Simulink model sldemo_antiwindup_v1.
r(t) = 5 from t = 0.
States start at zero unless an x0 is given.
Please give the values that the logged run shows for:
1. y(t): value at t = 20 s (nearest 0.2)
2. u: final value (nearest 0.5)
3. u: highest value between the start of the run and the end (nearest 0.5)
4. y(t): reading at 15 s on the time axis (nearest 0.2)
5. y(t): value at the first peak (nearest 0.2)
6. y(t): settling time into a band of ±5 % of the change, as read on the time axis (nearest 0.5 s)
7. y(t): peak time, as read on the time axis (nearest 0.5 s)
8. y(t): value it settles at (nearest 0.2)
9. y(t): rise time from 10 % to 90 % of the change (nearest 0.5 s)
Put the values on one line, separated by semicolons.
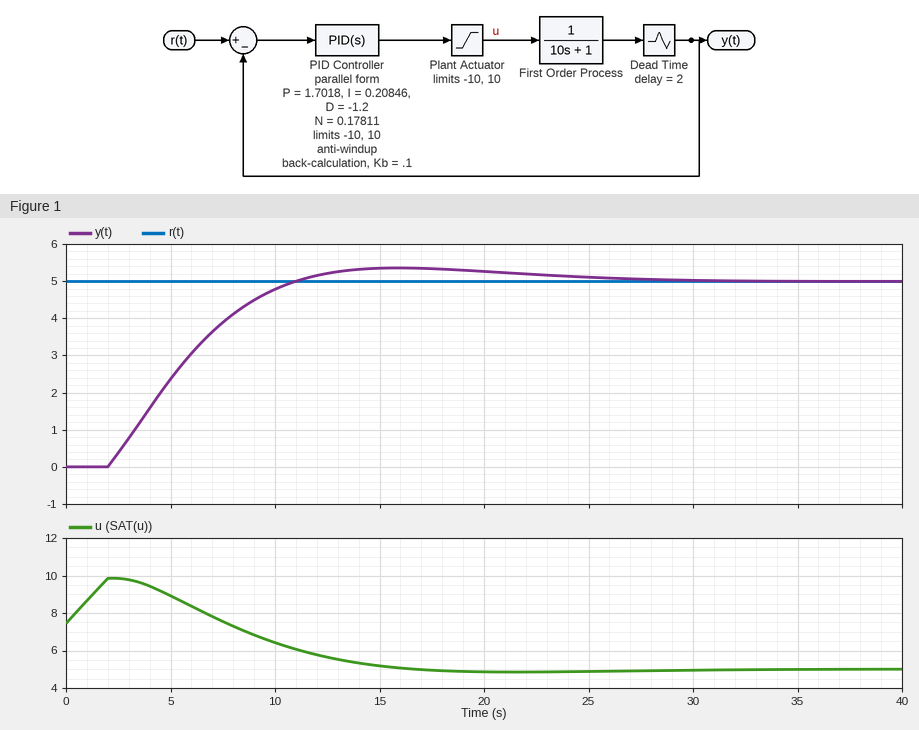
5.2; 5.0; 10.0; 5.4; 5.4; 20.5 s; 16.0 s; 5.0; 6.5 s
